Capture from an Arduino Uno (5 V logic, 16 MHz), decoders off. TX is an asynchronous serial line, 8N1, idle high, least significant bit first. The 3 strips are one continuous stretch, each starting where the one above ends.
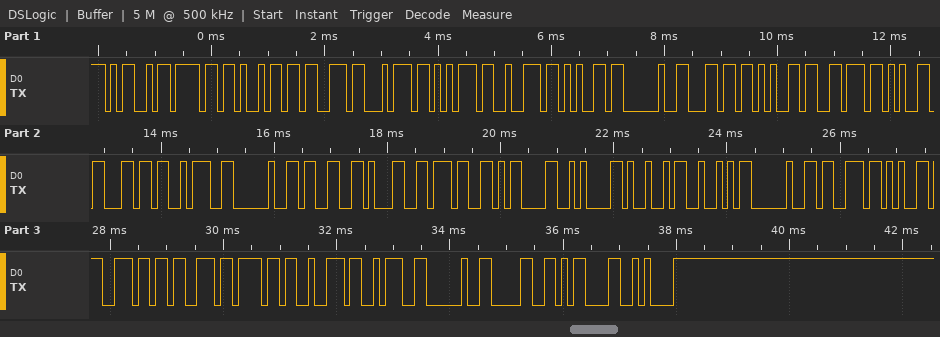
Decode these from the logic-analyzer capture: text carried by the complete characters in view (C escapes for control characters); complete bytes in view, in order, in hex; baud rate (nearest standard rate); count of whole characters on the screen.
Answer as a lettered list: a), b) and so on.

a) "Moisture level: 317\r\nIR sensor: 0\r\n"
b) 4D 6F 69 73 74 75 72 65 20 6C 65 76 65 6C 3A 20 33 31 37 0D 0A 49 52 20 73 65 6E 73 6F 72 3A 20 30 0D 0A
c) 9600 baud
d) 35
